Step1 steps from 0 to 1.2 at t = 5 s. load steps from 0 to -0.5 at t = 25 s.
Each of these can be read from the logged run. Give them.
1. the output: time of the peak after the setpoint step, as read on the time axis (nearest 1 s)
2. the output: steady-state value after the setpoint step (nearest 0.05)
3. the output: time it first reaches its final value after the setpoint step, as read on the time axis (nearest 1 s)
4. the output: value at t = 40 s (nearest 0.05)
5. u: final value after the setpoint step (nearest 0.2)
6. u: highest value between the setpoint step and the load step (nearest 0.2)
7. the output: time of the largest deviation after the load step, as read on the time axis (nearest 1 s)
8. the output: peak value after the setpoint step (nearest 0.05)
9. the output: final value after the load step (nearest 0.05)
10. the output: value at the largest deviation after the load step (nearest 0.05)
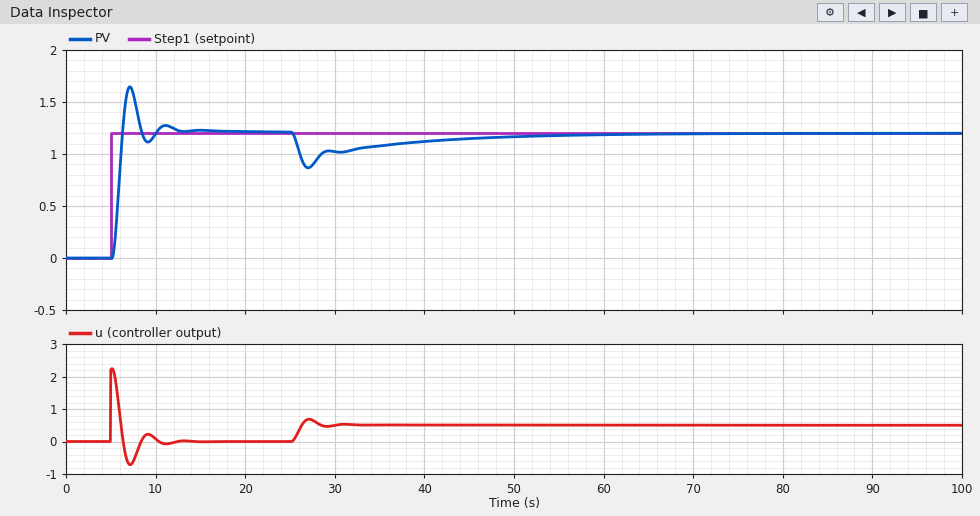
7 s
1.20
6 s
1.10
0.0
2.2
27 s
1.65
1.20
0.85
